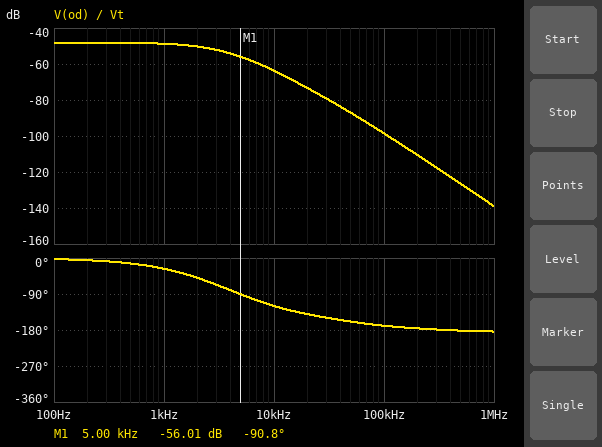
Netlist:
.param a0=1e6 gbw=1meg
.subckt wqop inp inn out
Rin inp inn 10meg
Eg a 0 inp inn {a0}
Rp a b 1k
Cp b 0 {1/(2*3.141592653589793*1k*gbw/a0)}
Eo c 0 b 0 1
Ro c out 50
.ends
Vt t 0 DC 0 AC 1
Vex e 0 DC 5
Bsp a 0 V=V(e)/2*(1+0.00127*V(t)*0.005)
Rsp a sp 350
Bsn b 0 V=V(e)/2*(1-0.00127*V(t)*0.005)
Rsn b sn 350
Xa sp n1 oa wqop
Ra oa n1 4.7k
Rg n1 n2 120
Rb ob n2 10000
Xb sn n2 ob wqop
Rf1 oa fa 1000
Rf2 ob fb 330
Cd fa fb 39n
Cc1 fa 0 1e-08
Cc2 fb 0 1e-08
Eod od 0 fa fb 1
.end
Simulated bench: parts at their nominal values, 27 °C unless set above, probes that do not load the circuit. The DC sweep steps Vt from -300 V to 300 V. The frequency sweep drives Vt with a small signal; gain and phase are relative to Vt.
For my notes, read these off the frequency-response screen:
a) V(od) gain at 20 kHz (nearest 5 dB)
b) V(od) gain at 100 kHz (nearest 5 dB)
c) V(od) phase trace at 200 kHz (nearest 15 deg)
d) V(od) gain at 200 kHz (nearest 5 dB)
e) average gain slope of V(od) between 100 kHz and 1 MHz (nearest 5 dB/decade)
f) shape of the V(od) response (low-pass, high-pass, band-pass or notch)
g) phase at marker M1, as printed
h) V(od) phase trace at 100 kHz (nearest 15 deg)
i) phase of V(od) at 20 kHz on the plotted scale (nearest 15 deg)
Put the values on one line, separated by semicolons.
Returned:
-75 dB; -100 dB; -180 deg; -110 dB; -40 dB/decade; low-pass; -90.8 deg; -165 deg; -135 deg
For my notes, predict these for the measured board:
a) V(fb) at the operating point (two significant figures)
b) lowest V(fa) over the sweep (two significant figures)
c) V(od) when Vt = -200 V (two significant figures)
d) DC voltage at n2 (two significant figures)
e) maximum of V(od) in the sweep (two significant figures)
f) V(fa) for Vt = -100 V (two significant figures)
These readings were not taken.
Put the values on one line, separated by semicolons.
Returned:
2.5 V; 2.1 V; -780 mV; 2.5 V; 1.2 V; 2.4 V
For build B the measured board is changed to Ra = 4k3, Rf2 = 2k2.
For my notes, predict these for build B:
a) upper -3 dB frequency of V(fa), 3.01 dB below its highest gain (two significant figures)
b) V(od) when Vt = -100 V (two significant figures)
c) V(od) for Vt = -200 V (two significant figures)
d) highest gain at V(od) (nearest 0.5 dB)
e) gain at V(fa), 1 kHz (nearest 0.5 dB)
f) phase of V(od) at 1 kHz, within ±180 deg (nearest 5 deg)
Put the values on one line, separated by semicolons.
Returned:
1.1 kHz; -380 mV; -760 mV; -48.5 dB; -61.5 dB; -50 deg
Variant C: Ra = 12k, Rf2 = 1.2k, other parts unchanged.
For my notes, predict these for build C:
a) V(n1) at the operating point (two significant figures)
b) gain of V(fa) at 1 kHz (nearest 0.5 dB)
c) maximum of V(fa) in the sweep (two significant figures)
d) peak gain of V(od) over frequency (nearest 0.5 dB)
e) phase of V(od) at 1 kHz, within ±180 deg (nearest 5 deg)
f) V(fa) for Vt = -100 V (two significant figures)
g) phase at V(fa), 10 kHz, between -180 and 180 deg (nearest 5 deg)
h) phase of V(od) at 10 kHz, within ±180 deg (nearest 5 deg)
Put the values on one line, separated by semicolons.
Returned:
2.5 V; -51.5 dB; 3.5 V; -44.5 dB; -40 deg; 2.2 V; -120 deg; -145 deg
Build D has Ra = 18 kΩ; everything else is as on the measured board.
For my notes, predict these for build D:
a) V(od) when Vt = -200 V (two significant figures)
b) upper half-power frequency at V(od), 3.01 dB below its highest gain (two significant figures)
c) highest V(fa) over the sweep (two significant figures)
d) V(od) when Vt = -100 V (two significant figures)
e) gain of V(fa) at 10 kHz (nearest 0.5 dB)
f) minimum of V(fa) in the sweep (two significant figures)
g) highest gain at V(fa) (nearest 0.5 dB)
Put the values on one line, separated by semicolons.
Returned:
-1.5 V; 2.1 kHz; 3.9 V; -740 mV; -66.5 dB; 1.1 V; -46.5 dB
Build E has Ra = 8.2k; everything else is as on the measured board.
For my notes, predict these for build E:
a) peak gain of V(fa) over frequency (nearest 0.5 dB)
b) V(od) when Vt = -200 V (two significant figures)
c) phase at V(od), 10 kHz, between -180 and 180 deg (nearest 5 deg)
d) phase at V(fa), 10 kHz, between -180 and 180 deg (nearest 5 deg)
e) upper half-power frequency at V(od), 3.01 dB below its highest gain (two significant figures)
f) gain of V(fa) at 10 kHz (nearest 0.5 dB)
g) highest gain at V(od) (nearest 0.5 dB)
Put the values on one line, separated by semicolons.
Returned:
-53.0 dB; -970 mV; -130 deg; 145 deg; 2.4 kHz; -64.0 dB; -46.5 dB
